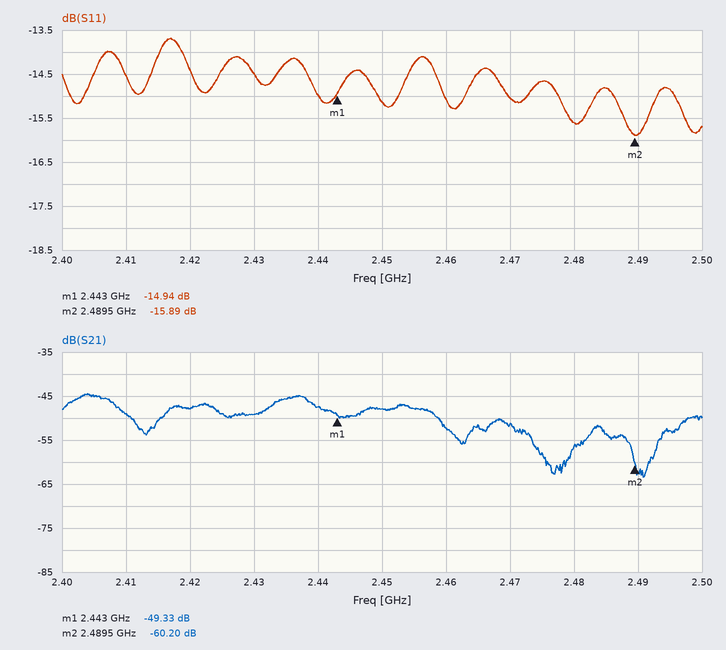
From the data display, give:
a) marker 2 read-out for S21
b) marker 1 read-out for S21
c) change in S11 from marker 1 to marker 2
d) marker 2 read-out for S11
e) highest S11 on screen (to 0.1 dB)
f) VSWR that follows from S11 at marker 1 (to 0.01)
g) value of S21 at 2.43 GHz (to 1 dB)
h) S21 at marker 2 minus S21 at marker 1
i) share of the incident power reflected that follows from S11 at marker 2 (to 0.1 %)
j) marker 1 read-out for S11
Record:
-60.20 dB
-49.33 dB
-0.95 dB
-15.89 dB
-13.7 dB
1.44
-49 dB
-10.87 dB
2.6 %
-14.94 dB
